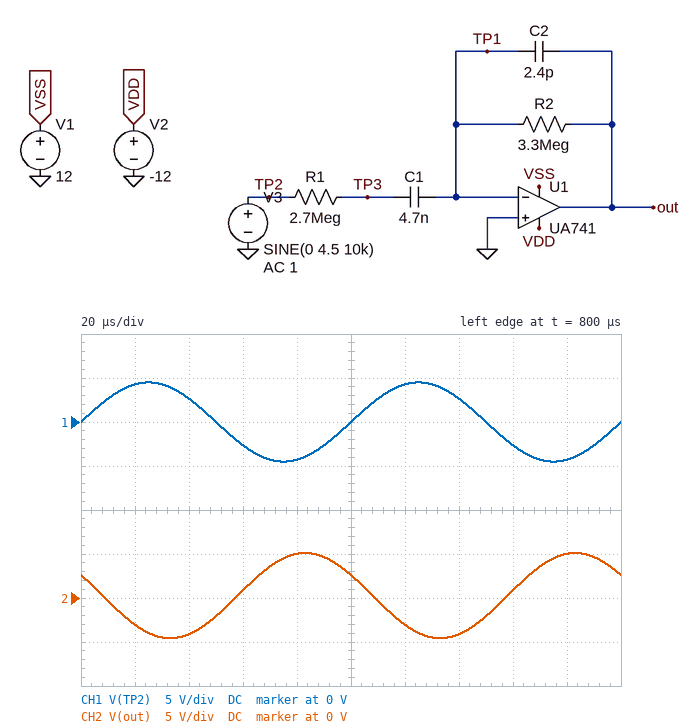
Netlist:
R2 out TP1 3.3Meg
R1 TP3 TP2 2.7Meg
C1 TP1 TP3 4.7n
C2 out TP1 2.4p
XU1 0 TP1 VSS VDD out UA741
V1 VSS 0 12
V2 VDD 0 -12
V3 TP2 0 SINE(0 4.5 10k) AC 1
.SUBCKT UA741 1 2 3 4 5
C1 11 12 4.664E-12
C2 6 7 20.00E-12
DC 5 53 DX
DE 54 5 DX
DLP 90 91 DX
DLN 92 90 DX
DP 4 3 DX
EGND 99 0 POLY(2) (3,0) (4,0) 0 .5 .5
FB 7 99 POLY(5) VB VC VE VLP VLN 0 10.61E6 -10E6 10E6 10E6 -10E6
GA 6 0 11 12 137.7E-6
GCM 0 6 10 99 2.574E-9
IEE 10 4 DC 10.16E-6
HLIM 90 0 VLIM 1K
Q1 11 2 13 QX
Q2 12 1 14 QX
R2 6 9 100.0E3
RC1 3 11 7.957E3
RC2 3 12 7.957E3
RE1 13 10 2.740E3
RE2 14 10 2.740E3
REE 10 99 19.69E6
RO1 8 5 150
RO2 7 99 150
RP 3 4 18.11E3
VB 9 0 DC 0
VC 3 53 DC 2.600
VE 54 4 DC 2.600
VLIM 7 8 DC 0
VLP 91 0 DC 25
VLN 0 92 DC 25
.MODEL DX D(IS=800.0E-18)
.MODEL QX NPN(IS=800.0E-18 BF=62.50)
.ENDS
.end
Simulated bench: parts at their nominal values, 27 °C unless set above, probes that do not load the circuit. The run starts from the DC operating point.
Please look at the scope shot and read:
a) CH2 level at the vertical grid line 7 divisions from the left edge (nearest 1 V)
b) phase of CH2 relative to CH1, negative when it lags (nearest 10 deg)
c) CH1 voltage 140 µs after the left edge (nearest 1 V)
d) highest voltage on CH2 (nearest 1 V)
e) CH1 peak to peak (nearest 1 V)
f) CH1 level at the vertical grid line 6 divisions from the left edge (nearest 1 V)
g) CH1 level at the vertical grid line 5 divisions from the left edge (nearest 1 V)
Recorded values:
-4 V
150 deg
3 V
5 V
9 V
4 V
0 V
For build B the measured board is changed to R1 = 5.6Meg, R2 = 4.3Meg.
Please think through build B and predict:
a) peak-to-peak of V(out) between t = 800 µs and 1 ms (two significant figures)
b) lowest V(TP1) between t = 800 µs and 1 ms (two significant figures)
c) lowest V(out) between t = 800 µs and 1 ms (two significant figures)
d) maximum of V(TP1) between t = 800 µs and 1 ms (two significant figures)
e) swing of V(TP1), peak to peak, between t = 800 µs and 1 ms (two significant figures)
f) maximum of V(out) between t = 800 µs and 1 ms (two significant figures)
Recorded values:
5.7 V
-27 mV
-2.5 V
27 mV
53 mV
3.2 V
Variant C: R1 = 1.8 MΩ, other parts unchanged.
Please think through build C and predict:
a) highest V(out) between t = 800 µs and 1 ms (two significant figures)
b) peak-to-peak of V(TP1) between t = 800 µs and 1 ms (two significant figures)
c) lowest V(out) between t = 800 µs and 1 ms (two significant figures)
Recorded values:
7.5 V
170 mV
-7.0 V
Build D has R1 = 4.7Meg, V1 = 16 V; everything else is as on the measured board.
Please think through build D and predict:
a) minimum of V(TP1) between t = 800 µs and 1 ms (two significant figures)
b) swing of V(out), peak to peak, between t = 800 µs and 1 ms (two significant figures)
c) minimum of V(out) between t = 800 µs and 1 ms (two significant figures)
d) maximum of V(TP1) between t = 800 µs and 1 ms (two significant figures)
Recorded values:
-26 mV
5.6 V
-2.5 V
26 mV
